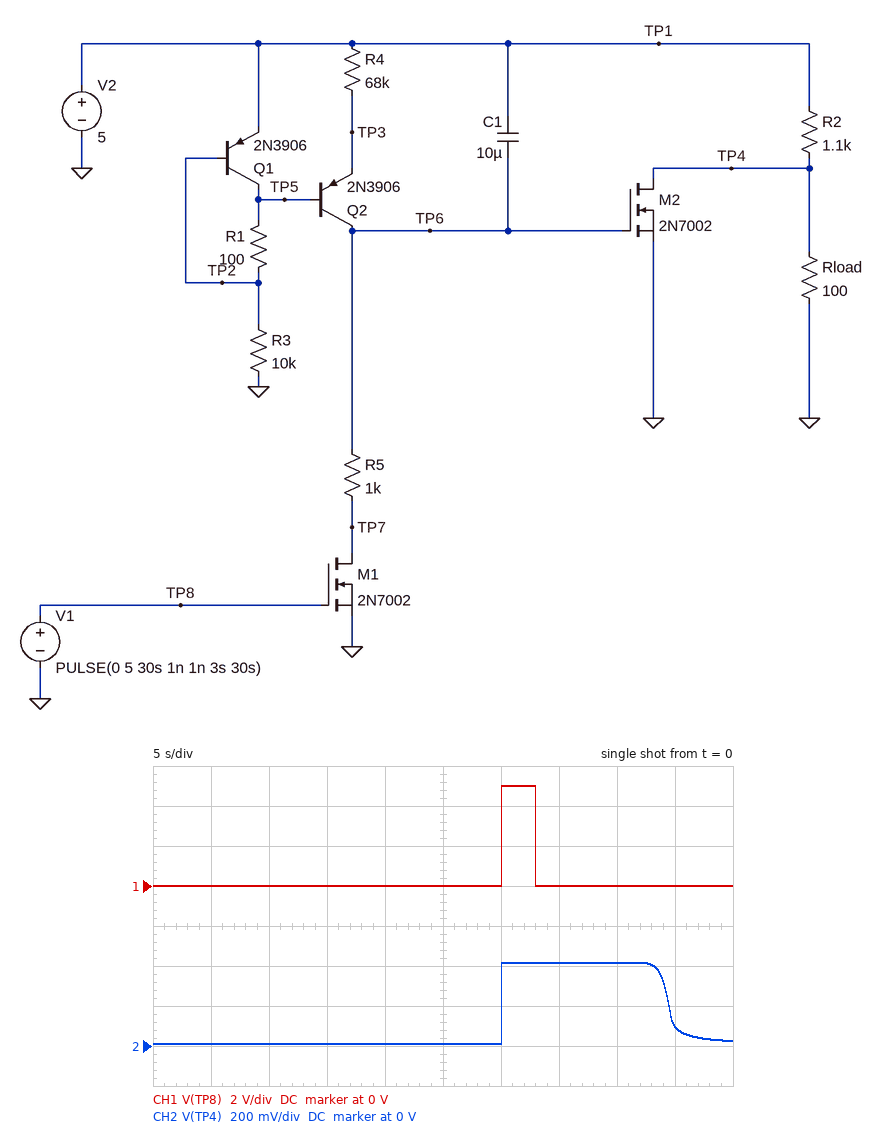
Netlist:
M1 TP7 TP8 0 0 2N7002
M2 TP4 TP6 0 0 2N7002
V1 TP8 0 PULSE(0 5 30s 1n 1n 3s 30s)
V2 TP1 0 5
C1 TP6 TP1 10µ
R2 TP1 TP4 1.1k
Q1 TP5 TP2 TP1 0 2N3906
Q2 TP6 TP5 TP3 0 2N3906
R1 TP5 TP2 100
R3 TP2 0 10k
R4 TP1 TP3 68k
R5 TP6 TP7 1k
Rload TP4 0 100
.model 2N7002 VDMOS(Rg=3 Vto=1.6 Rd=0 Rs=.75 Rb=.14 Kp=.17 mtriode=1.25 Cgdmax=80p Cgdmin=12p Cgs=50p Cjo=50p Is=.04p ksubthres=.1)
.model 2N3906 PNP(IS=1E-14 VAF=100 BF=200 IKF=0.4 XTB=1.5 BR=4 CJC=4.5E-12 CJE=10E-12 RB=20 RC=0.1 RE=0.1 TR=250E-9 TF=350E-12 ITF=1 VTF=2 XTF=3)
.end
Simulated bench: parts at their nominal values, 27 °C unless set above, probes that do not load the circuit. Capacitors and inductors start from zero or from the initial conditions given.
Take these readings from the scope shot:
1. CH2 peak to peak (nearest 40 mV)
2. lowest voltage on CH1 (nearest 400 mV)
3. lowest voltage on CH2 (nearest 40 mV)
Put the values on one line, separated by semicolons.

400 mV; 0 V; 0 V
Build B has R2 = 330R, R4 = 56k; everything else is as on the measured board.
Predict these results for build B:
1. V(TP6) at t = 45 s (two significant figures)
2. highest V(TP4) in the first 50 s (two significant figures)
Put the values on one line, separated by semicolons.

2.1 V; 1.2 V
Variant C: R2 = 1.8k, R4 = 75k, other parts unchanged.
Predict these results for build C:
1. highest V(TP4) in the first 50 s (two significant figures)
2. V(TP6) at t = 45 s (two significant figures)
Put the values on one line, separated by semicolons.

260 mV; 1.7 V
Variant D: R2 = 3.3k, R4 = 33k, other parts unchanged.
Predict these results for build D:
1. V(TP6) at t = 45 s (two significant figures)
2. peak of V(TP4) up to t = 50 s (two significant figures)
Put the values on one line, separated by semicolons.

3.2 V; 150 mV
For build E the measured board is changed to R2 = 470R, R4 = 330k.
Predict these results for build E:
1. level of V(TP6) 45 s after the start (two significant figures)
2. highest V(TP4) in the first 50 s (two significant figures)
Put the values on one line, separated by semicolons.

500 mV; 880 mV
